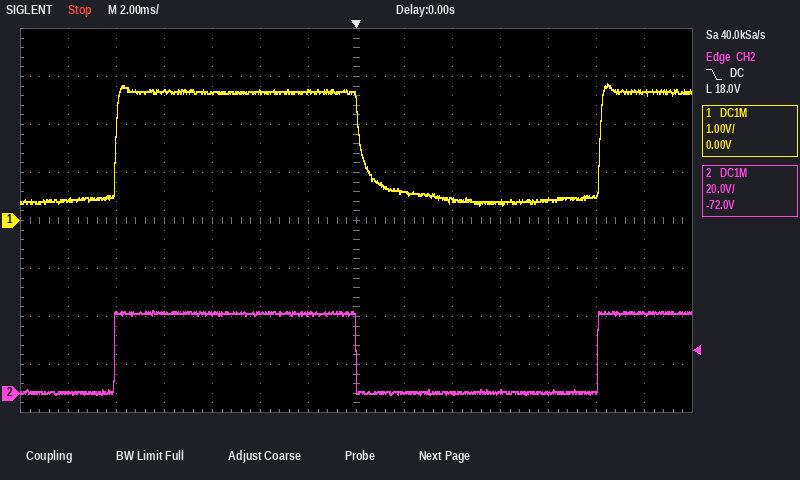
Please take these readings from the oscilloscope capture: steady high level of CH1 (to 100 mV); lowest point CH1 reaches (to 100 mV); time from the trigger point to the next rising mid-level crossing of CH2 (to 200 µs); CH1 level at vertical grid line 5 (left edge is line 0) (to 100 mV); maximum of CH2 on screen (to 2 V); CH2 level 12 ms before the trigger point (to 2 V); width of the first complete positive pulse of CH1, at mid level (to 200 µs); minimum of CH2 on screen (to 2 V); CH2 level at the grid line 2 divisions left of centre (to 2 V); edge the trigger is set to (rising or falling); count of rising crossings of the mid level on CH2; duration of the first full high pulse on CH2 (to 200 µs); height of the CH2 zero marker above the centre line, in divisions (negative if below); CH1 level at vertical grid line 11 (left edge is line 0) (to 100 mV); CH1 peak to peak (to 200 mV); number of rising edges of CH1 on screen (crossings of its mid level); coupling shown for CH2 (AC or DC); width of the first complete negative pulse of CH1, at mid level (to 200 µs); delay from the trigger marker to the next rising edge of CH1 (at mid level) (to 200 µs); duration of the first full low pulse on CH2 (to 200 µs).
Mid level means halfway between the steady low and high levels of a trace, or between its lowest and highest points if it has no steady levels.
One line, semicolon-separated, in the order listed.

2.7 V; 300 mV; 10.0 ms; 2.7 V; 34 V; 0 V; 10.2 ms; 0 V; 34 V; falling; 2; 10.0 ms; -3.6 div; 400 mV; 2.6 V; 2; DC; 10.0 ms; 10.2 ms; 10.0 ms
